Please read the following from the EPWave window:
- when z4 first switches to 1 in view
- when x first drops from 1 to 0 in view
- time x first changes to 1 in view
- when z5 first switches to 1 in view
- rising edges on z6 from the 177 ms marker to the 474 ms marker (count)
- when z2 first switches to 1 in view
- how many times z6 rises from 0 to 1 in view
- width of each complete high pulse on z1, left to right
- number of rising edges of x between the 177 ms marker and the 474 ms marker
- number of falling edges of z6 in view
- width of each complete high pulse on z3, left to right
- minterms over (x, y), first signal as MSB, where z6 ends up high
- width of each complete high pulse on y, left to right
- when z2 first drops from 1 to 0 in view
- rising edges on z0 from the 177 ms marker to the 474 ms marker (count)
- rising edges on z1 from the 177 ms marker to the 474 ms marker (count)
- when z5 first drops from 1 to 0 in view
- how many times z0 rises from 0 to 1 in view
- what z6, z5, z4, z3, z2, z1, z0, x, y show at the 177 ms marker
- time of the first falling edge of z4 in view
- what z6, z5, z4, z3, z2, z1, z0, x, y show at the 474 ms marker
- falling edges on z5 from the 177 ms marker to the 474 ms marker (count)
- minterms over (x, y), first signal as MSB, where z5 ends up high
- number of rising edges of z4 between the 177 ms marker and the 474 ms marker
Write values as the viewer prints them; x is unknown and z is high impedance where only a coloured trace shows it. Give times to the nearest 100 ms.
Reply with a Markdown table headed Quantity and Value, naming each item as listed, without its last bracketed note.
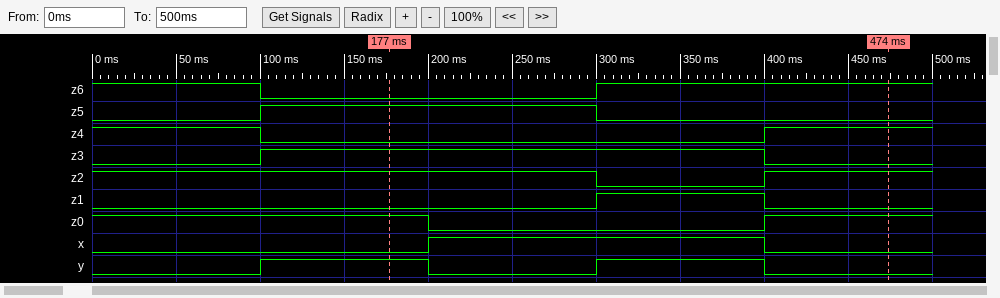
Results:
| Quantity | Value |
|---|---|
| when z4 first switches to 1 in view | 400 ms |
| when x first drops from 1 to 0 in view | 400 ms |
| time x first changes to 1 in view | 200 ms |
| when z5 first switches to 1 in view | 100 ms |
| rising edges on z6 from the 177 ms marker to the 474 ms marker | 1 |
| when z2 first switches to 1 in view | 400 ms |
| how many times z6 rises from 0 to 1 in view | 1 |
| width of each complete high pulse on z1, left to right | 100 ms |
| number of rising edges of x between the 177 ms marker and the 474 ms marker | 1 |
| number of falling edges of z6 in view | 1 |
| width of each complete high pulse on z3, left to right | 300 ms |
| minterms over (x, y), first signal as MSB, where z6 ends up high | 0, 3 |
| width of each complete high pulse on y, left to right | 100 ms, 100 ms |
| when z2 first drops from 1 to 0 in view | 300 ms |
| rising edges on z0 from the 177 ms marker to the 474 ms marker | 1 |
| rising edges on z1 from the 177 ms marker to the 474 ms marker | 1 |
| when z5 first drops from 1 to 0 in view | 300 ms |
| how many times z0 rises from 0 to 1 in view | 1 |
| what z6, z5, z4, z3, z2, z1, z0, x, y show at the 177 ms marker | z6=0, z5=1, z4=0, z3=1, z2=1, z1=0, z0=1, x=0, y=1 |
| time of the first falling edge of z4 in view | 100 ms |
| what z6, z5, z4, z3, z2, z1, z0, x, y show at the 474 ms marker | z6=1, z5=0, z4=1, z3=0, z2=1, z1=0, z0=1, x=0, y=0 |
| falling edges on z5 from the 177 ms marker to the 474 ms marker | 1 |
| minterms over (x, y), first signal as MSB, where z5 ends up high | 1, 2 |
| number of rising edges of z4 between the 177 ms marker and the 474 ms marker | 1 |
